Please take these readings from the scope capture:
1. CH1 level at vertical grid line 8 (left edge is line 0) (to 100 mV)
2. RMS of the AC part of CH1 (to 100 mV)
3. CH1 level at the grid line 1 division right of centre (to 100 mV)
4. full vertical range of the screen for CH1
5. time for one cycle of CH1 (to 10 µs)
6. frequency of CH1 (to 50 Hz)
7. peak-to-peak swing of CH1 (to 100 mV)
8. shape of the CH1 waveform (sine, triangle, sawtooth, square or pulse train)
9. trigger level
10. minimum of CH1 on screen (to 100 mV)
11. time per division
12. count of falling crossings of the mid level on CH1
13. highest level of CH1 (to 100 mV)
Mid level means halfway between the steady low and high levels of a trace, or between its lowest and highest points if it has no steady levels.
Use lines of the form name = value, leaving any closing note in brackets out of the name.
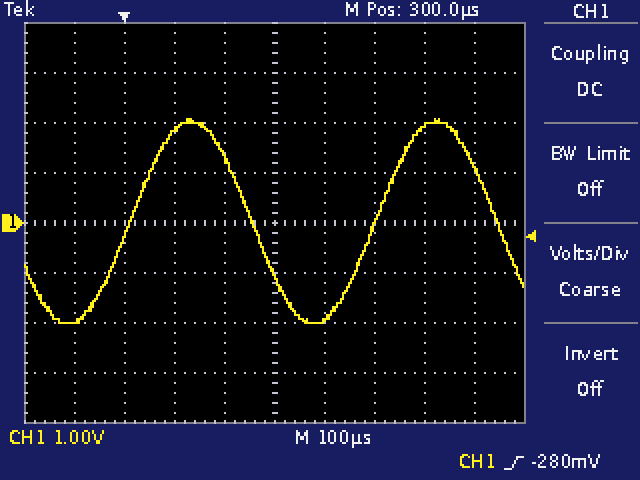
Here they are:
CH1 level at vertical grid line 8 (left edge is line 0) = 1.9 V
RMS of the AC part of CH1 = 1.4 V
CH1 level at the grid line 1 division right of centre = -1.9 V
full vertical range of the screen for CH1 = 8 V
time for one cycle of CH1 = 490 µs
frequency of CH1 = 2.05 kHz
peak-to-peak swing of CH1 = 4.1 V
shape of the CH1 waveform = sine
trigger level = -280 mV
minimum of CH1 on screen = -2.0 V
time per division = 100 µs
count of falling crossings of the mid level on CH1 = 2
highest level of CH1 = 2.1 V
